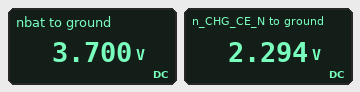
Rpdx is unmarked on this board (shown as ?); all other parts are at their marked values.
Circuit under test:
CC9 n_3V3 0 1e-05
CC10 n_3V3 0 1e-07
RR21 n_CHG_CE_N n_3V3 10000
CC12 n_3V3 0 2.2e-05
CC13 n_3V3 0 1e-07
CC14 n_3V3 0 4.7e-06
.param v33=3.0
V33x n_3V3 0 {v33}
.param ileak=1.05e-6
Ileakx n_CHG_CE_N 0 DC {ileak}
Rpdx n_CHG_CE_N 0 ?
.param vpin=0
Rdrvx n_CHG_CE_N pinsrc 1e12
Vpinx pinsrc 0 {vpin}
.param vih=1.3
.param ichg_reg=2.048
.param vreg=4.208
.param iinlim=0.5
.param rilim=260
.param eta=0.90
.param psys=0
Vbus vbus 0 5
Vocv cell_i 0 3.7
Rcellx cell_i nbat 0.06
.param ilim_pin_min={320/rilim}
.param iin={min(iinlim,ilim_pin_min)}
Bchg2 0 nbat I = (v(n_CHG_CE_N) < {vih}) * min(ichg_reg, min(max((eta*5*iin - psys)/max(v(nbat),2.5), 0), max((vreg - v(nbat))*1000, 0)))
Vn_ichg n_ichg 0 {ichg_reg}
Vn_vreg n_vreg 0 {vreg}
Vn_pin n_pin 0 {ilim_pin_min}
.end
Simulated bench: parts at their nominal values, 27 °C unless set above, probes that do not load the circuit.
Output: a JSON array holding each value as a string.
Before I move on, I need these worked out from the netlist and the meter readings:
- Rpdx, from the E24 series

["33 kΩ"]
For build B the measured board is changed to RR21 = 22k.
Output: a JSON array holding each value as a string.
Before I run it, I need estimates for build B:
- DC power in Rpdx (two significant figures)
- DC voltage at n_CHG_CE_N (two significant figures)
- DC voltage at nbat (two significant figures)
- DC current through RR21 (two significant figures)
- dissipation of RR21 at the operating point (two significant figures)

["97 µW", "1.8 V", "3.7 V", "55 µA", "67 µW"]
